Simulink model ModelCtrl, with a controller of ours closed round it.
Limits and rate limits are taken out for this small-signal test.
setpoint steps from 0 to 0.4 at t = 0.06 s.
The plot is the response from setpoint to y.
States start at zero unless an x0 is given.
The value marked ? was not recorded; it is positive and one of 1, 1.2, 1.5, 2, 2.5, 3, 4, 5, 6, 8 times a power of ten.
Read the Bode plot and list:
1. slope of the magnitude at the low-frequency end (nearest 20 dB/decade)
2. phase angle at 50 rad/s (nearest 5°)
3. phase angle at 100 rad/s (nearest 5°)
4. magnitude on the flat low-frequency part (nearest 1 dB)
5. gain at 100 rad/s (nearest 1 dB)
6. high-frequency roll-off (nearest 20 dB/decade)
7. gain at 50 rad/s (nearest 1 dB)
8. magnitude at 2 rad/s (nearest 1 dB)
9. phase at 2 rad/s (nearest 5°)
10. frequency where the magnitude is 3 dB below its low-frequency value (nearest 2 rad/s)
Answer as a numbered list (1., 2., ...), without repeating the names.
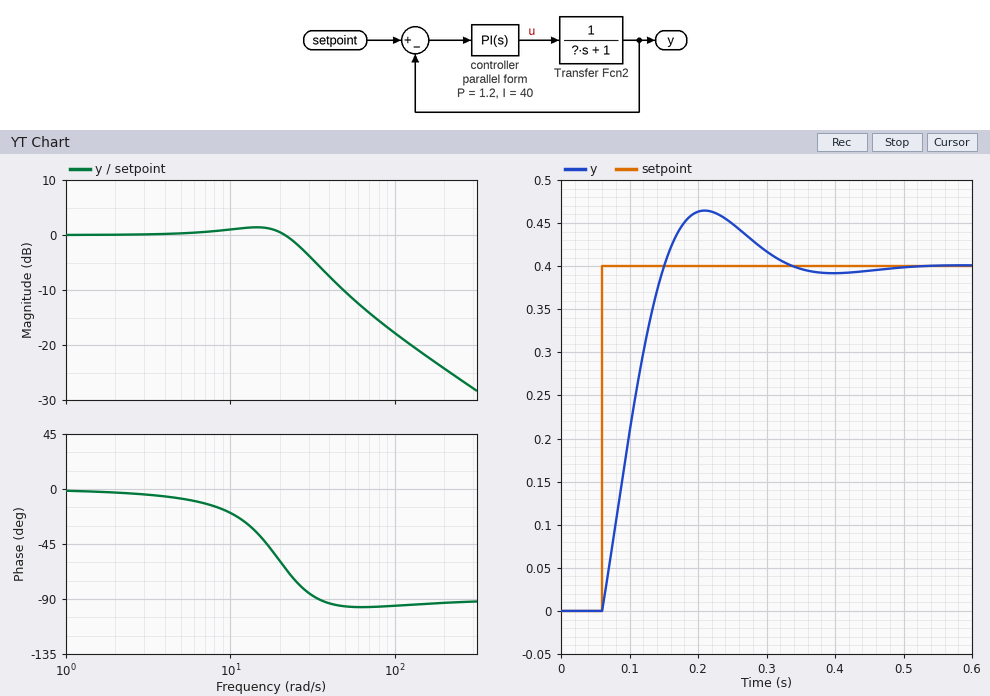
1. 0 dB/decade
2. -95°
3. -95°
4. 0 dB
5. -18 dB
6. -20 dB/decade
7. -10 dB
8. 0 dB
9. -5°
10. 28 rad/s
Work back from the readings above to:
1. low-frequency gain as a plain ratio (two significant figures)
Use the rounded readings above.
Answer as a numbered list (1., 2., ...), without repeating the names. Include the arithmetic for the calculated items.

1. 10^(0 / 20) = 1.0
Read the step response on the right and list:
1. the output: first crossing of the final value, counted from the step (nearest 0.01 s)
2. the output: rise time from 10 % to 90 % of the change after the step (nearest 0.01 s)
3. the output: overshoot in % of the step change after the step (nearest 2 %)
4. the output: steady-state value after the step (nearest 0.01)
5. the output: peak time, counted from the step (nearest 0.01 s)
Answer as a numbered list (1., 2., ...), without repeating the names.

1. 0.09 s
2. 0.07 s
3. 16 %
4. 0.40
5. 0.15 s
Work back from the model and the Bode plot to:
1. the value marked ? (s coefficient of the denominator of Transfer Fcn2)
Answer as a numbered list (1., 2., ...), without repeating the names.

1. 0.1
